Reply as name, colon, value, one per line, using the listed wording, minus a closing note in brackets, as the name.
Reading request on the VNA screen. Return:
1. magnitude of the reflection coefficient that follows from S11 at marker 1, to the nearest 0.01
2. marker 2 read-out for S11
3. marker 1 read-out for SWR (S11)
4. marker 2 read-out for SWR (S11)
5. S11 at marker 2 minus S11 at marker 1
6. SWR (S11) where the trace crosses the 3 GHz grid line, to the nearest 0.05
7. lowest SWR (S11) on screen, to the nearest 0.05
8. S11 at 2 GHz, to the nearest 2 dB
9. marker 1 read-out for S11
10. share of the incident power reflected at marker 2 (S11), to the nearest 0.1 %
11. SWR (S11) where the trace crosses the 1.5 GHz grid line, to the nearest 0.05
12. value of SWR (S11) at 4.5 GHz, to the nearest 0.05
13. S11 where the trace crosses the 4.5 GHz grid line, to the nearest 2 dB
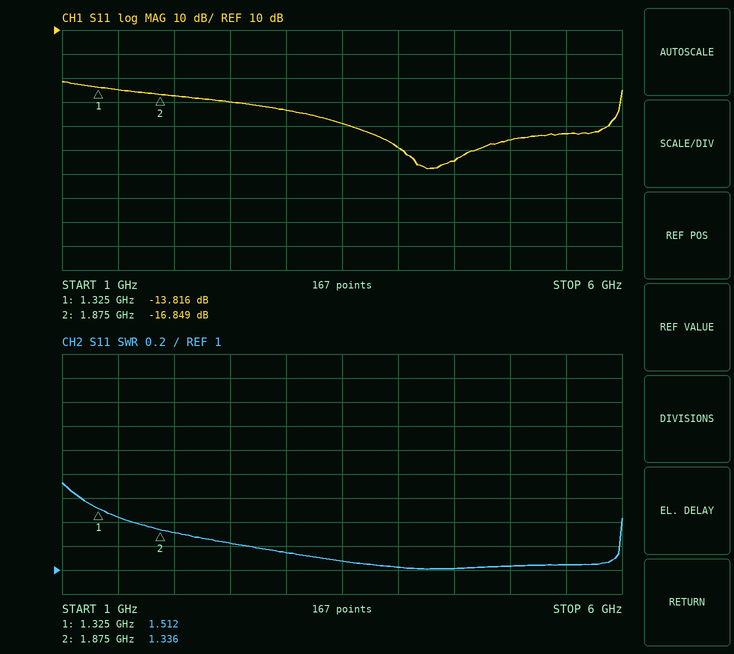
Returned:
magnitude of the reflection coefficient that follows from S11 at marker 1, to the nearest 0.01: 0.20
marker 2 read-out for S11: -16.849 dB
marker 1 read-out for SWR: 1.512
marker 2 read-out for SWR: 1.336
S11 at marker 2 minus S11 at marker 1: -3.033 dB
SWR (S11) where the trace crosses the 3 GHz grid line, to the nearest 0.05: 1.15
lowest SWR (S11) on screen, to the nearest 0.05: 1.00
S11 at 2 GHz, to the nearest 2 dB: -18 dB
marker 1 read-out for S11: -13.816 dB
share of the incident power reflected at marker 2 (S11), to the nearest 0.1 %: 2.1 %
SWR (S11) where the trace crosses the 1.5 GHz grid line, to the nearest 0.05: 1.45
value of SWR (S11) at 4.5 GHz, to the nearest 0.05: 1.00
S11 where the trace crosses the 4.5 GHz grid line, to the nearest 2 dB: -44 dB
